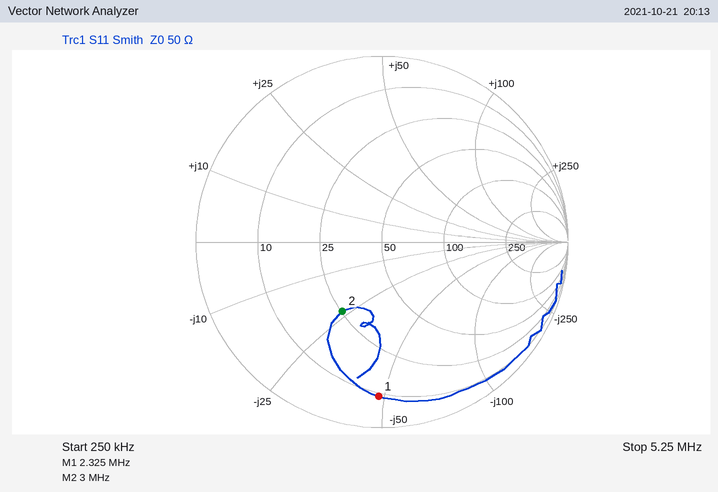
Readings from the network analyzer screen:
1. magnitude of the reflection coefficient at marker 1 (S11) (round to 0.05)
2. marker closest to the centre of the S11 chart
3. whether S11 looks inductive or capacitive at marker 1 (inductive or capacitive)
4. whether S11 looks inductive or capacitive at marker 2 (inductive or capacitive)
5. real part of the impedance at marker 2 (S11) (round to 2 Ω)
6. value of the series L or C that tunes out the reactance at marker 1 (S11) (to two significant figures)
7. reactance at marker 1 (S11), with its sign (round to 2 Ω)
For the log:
0.85
marker 2
capacitive
capacitive
26 Ω
3.3 µH
-48 Ω
